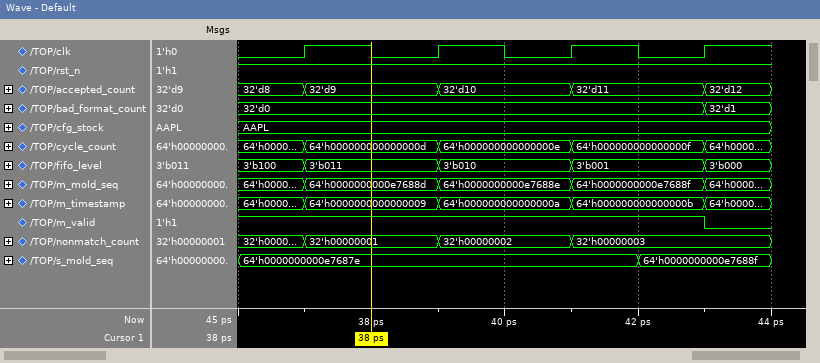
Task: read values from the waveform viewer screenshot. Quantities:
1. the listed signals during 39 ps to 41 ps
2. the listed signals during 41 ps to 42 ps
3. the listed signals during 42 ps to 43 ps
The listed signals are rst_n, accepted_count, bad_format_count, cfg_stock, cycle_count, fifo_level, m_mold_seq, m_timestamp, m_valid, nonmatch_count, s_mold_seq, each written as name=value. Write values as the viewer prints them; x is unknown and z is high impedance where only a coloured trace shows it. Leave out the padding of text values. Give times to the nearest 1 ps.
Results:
rst_n=1, accepted_count=32'd10, bad_format_count=32'd0, cfg_stock=AAPL, cycle_count=64'h000000000000000e, fifo_level=3'b010, m_mold_seq=64'h0000000000e7688e, m_timestamp=64'h000000000000000a, m_valid=1, nonmatch_count=32'h00000002, s_mold_seq=64'h0000000000e7687e
rst_n=1, accepted_count=32'd11, bad_format_count=32'd0, cfg_stock=AAPL, cycle_count=64'h000000000000000f, fifo_level=3'b001, m_mold_seq=64'h0000000000e7688f, m_timestamp=64'h000000000000000b, m_valid=1, nonmatch_count=32'h00000003, s_mold_seq=64'h0000000000e7687e
rst_n=1, accepted_count=32'd11, bad_format_count=32'd0, cfg_stock=AAPL, cycle_count=64'h000000000000000f, fifo_level=3'b001, m_mold_seq=64'h0000000000e7688f, m_timestamp=64'h000000000000000b, m_valid=1, nonmatch_count=32'h00000003, s_mold_seq=64'h0000000000e7688f
